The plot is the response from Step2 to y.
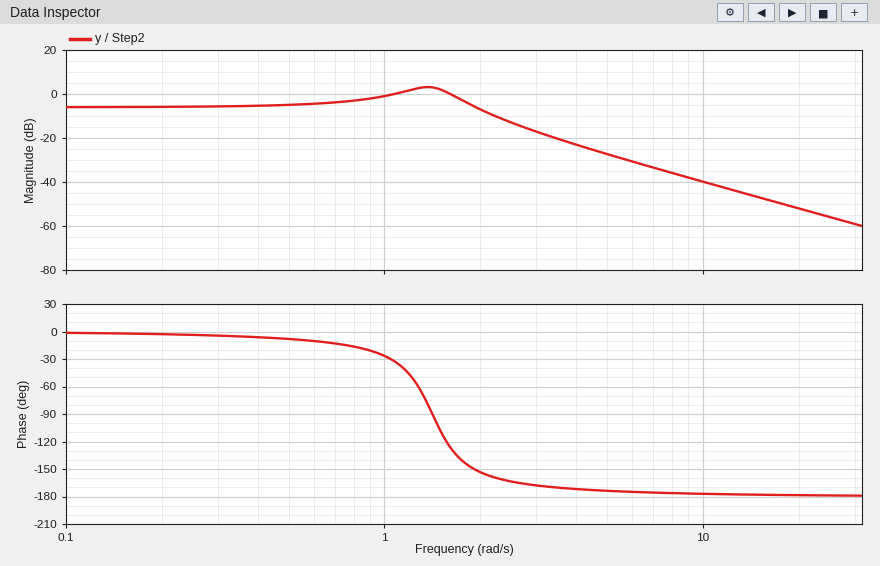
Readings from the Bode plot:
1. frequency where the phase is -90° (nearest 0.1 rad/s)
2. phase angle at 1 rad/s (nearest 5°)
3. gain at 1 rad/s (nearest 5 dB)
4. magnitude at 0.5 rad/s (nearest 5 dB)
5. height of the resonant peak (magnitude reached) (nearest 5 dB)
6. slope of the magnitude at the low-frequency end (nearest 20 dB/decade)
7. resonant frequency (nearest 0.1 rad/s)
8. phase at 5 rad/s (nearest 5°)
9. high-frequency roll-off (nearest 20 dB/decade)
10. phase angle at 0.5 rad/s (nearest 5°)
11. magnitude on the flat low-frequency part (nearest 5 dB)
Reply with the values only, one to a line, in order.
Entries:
1.4 rad/s
-25°
0 dB
-5 dB
5 dB
0 dB/decade
1.4 rad/s
-175°
-40 dB/decade
-10°
-5 dB
